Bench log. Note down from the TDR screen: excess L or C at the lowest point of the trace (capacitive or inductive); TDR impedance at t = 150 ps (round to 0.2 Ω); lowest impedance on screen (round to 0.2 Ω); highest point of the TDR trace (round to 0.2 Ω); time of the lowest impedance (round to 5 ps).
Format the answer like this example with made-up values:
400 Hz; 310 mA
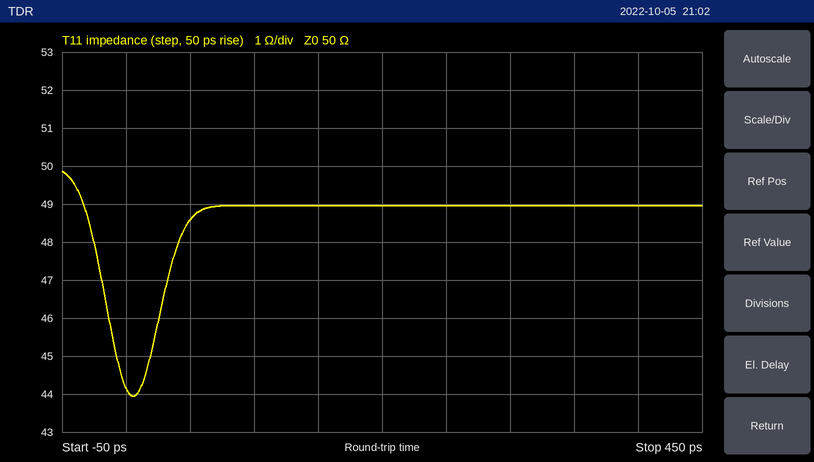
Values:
capacitive; 49.0 Ω; 44.0 Ω; 49.8 Ω; 5 ps
